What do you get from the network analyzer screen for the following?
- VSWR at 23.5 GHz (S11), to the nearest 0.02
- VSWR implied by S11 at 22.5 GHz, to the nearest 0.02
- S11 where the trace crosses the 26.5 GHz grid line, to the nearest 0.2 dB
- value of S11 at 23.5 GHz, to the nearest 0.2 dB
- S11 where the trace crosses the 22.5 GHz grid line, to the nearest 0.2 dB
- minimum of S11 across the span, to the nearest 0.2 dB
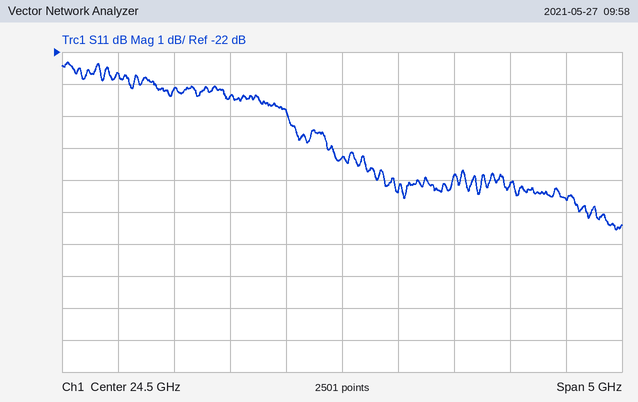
1.14
1.16
-26.6 dB
-23.4 dB
-22.6 dB
-27.6 dB
